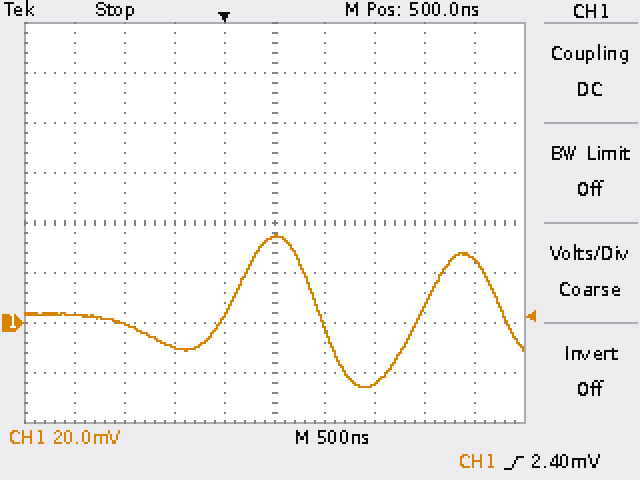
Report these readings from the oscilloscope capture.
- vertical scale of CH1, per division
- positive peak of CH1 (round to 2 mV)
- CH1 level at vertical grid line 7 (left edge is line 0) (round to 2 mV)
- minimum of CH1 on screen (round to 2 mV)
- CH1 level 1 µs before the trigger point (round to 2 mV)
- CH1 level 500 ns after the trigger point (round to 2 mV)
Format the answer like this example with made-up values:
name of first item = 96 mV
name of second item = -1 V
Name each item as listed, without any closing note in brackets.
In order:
vertical scale of CH1, per division = 20 mV
positive peak of CH1 = 36 mV
CH1 level at vertical grid line 7 (left edge is line 0) = -24 mV
minimum of CH1 on screen = -26 mV
CH1 level 1 µs before the trigger point = 0 mV
CH1 level 500 ns after the trigger point = 34 mV
